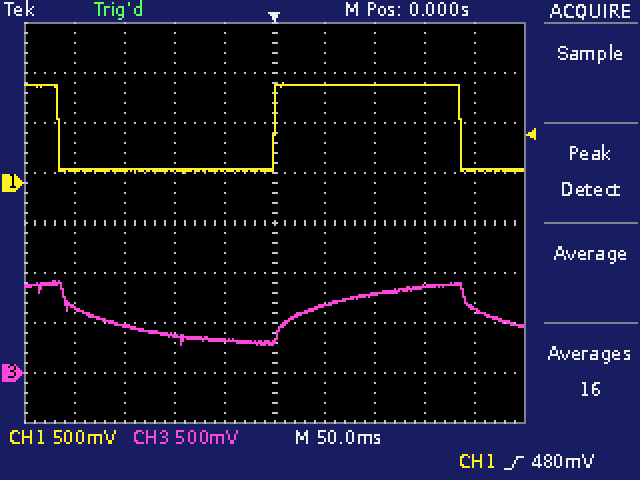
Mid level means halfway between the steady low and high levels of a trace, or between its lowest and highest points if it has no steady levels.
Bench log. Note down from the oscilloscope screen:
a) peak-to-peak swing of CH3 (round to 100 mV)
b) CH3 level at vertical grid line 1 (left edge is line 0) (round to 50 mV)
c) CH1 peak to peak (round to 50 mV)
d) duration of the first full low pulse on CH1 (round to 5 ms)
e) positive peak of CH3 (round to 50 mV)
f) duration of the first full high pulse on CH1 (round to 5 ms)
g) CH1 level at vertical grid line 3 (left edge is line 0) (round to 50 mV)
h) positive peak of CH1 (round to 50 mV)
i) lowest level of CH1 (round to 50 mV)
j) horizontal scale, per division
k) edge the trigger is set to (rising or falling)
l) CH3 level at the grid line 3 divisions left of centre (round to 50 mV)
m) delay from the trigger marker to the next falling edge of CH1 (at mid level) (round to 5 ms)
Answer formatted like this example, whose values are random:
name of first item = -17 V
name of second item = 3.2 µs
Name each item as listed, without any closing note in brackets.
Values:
peak-to-peak swing of CH3 = 600 mV
CH3 level at vertical grid line 1 (left edge is line 0) = 650 mV
CH1 peak to peak = 900 mV
duration of the first full low pulse on CH1 = 215 ms
positive peak of CH3 = 900 mV
duration of the first full high pulse on CH1 = 185 ms
CH1 level at vertical grid line 3 (left edge is line 0) = 150 mV
positive peak of CH1 = 1.00 V
lowest level of CH1 = 100 mV
horizontal scale, per division = 50 ms
edge the trigger is set to = rising
CH3 level at the grid line 3 divisions left of centre = 450 mV
delay from the trigger marker to the next falling edge of CH1 (at mid level) = 185 ms
